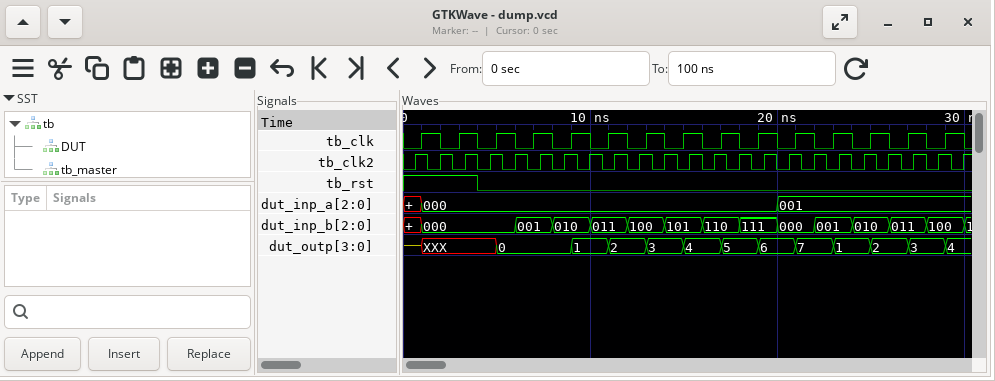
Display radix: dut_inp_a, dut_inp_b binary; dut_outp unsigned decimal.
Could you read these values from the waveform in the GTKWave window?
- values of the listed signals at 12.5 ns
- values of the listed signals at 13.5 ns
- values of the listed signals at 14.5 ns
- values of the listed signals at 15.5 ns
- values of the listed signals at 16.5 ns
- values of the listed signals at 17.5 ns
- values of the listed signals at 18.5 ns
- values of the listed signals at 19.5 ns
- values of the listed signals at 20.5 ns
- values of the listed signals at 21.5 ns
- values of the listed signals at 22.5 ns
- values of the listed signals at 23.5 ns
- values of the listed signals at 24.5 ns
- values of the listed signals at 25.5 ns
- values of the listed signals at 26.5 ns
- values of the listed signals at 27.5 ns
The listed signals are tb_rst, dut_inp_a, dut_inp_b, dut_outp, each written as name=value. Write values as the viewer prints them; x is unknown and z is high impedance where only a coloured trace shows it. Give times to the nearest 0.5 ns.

tb_rst=0, dut_inp_a=000, dut_inp_b=100, dut_outp=2
tb_rst=0, dut_inp_a=000, dut_inp_b=100, dut_outp=3
tb_rst=0, dut_inp_a=000, dut_inp_b=101, dut_outp=3
tb_rst=0, dut_inp_a=000, dut_inp_b=101, dut_outp=4
tb_rst=0, dut_inp_a=000, dut_inp_b=110, dut_outp=4
tb_rst=0, dut_inp_a=000, dut_inp_b=110, dut_outp=5
tb_rst=0, dut_inp_a=000, dut_inp_b=111, dut_outp=5
tb_rst=0, dut_inp_a=000, dut_inp_b=111, dut_outp=6
tb_rst=0, dut_inp_a=001, dut_inp_b=000, dut_outp=6
tb_rst=0, dut_inp_a=001, dut_inp_b=000, dut_outp=7
tb_rst=0, dut_inp_a=001, dut_inp_b=001, dut_outp=7
tb_rst=0, dut_inp_a=001, dut_inp_b=001, dut_outp=1
tb_rst=0, dut_inp_a=001, dut_inp_b=010, dut_outp=1
tb_rst=0, dut_inp_a=001, dut_inp_b=010, dut_outp=2
tb_rst=0, dut_inp_a=001, dut_inp_b=011, dut_outp=2
tb_rst=0, dut_inp_a=001, dut_inp_b=011, dut_outp=3
